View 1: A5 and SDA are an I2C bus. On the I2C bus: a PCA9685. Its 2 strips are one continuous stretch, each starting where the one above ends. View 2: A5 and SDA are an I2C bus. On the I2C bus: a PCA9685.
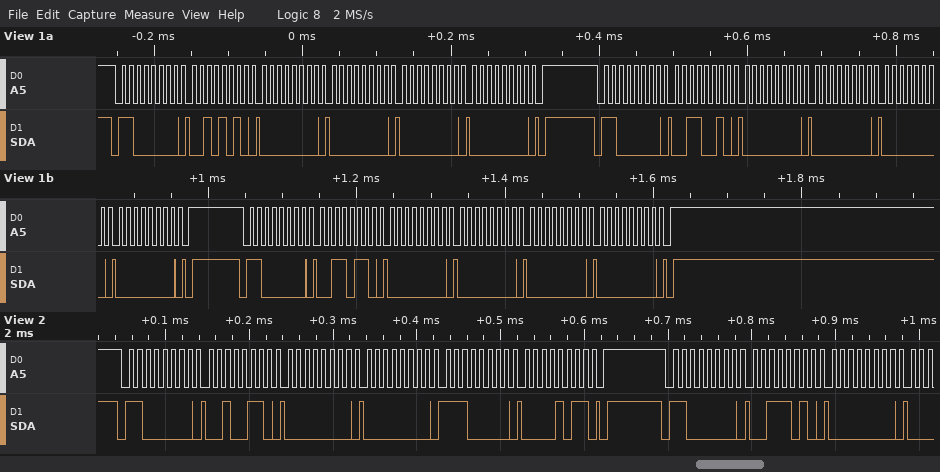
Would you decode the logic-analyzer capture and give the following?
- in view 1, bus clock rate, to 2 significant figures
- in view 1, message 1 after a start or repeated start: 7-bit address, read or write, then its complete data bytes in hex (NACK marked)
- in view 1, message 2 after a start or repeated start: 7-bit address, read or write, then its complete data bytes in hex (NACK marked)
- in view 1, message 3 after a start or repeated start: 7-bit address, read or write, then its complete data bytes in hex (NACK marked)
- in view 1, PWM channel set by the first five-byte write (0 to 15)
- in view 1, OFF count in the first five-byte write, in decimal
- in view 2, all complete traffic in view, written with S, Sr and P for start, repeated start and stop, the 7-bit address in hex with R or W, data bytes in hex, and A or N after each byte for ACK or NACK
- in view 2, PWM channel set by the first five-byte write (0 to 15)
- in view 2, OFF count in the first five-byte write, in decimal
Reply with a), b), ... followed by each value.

a) 100 kHz
b) 0x60 write: 2A 00 00 00 00
c) 0x60 write: 32 00 00 00 00
d) 0x60 write: 36 00 00 00 00
e) 9
f) 0
g) S 60W A 26 A 00 A 00 A E0 A 0B A P S 60W A 3A A 00 A
h) 8
i) 3040
